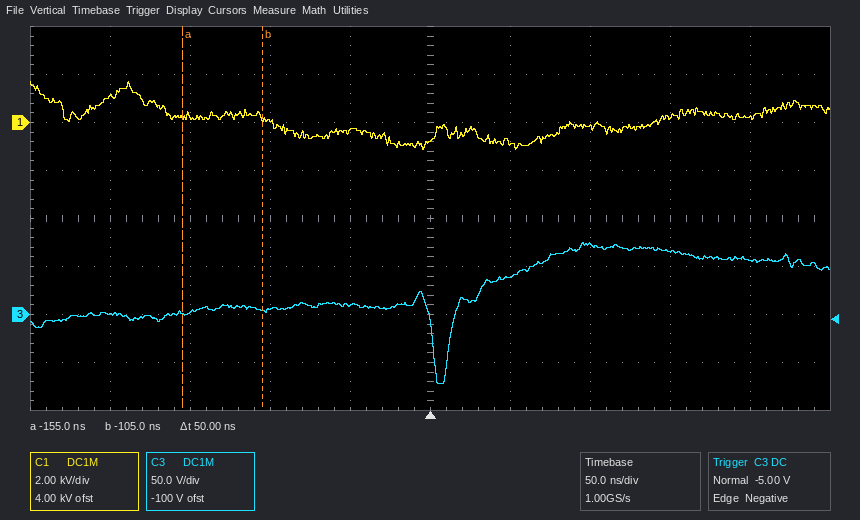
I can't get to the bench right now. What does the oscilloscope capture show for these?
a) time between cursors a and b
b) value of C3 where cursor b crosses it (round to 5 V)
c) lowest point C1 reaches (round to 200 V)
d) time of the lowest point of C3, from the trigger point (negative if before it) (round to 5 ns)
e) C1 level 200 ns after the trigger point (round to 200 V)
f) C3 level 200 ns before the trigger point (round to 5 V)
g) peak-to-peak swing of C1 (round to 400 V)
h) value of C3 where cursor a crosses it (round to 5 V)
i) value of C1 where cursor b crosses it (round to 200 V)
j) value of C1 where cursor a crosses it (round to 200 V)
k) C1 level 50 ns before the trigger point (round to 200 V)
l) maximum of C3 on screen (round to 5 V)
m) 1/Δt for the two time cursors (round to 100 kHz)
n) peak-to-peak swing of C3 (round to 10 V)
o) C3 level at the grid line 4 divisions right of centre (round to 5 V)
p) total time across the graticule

50 ns
5 V
-1.2 kV
+5 ns
200 V
0 V
2.8 kV
0 V
200 V
200 V
-400 V
75 V
20.0 MHz
150 V
55 V
500 ns
